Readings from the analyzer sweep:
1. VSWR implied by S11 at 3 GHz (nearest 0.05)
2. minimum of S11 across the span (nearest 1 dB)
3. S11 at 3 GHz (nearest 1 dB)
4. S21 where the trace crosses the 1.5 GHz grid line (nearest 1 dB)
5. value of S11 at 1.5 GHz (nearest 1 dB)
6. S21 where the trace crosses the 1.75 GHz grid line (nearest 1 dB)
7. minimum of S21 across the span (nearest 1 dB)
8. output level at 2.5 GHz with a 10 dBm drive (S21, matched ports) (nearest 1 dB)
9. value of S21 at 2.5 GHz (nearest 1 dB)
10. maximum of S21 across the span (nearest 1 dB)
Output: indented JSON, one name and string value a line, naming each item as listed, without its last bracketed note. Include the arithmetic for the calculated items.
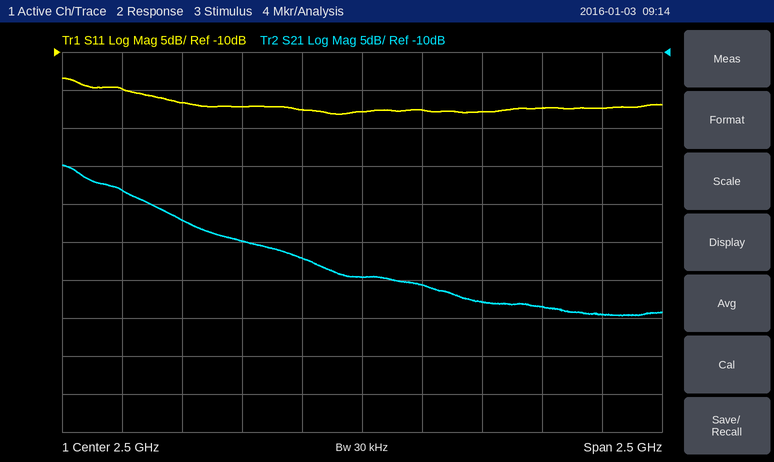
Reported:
{
  "VSWR implied by S11 at 3 GHz": "|Γ| = 10^(-18/20) = 0.1259; VSWR = (1 + 0.1259)/(1 − 0.1259) ≈ 1.29, so 1.30 to the nearest 0.05",
  "minimum of S11 across the span": "-18 dB",
  "S11 at 3 GHz": "-18 dB",
  "S21 where the trace crosses the 1.5 GHz grid line": "-28 dB",
  "value of S11 at 1.5 GHz": "-15 dB",
  "S21 where the trace crosses the 1.75 GHz grid line": "-32 dB",
  "minimum of S21 across the span": "-45 dB",
  "output level at 2.5 GHz with a 10 dBm drive (S21, matched ports)": "10 dBm + (-40 dB) = -30 dBm",
  "value of S21 at 2.5 GHz": "-40 dB",
  "maximum of S21 across the span": "-25 dB"
}
